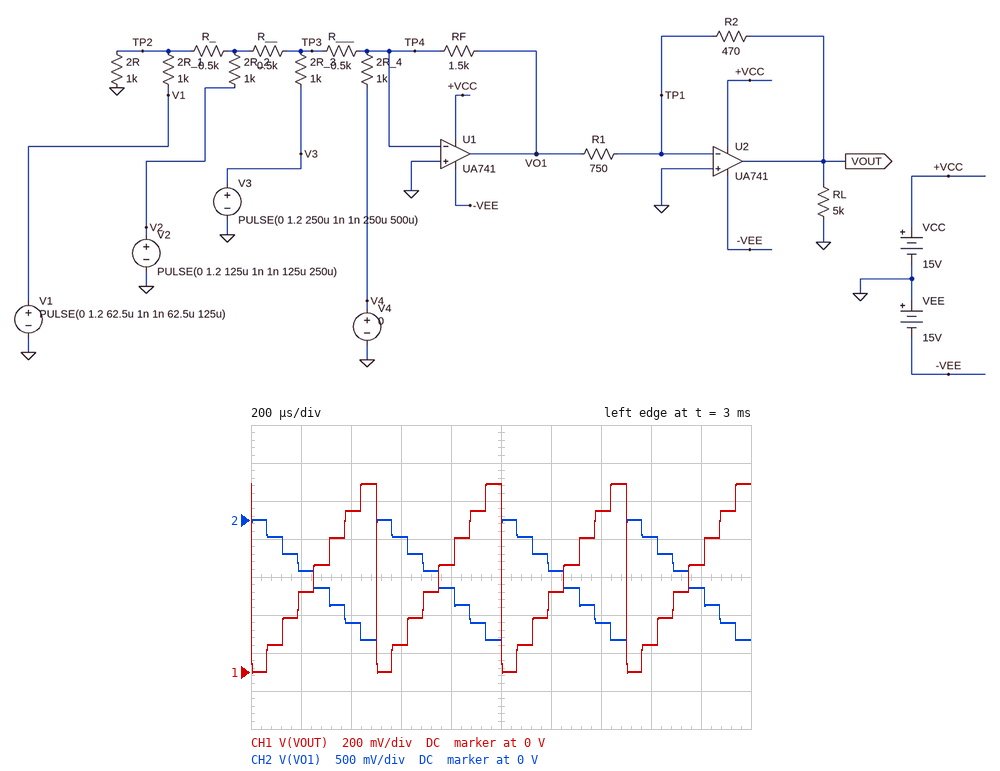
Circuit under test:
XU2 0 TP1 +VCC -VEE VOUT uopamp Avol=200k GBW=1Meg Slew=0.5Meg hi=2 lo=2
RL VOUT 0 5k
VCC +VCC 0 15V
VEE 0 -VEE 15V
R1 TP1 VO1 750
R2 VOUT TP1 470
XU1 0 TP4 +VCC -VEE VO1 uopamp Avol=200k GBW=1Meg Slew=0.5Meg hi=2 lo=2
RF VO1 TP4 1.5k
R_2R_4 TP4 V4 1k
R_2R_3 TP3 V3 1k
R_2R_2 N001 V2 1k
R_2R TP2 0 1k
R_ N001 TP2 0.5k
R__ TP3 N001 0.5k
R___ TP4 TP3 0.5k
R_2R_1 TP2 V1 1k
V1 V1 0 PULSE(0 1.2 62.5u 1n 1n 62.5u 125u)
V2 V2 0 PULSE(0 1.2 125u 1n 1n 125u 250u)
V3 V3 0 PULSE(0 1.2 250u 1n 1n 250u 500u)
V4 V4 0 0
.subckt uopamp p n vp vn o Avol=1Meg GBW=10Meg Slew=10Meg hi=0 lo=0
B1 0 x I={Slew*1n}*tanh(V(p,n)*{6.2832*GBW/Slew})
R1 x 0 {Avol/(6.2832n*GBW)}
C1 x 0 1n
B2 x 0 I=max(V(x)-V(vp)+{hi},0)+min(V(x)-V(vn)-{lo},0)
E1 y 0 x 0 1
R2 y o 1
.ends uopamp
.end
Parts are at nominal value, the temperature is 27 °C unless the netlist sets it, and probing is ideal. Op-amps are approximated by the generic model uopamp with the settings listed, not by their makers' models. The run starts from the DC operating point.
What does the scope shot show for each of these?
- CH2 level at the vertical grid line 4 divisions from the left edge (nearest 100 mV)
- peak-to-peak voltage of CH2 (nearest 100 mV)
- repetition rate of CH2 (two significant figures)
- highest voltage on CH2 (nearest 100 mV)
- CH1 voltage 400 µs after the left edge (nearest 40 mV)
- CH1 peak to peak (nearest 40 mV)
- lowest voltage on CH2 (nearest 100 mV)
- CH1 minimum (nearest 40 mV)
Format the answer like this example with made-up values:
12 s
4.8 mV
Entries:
-900 mV
1.6 V
2.0 kHz
0 V
840 mV
1.00 V
-1.6 V
0 V
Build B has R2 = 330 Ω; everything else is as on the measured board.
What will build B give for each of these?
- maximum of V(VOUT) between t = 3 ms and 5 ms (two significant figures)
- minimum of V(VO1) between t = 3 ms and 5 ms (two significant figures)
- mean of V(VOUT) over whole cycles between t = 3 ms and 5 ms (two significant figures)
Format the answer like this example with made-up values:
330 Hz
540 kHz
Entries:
690 mV
-1.6 V
350 mV
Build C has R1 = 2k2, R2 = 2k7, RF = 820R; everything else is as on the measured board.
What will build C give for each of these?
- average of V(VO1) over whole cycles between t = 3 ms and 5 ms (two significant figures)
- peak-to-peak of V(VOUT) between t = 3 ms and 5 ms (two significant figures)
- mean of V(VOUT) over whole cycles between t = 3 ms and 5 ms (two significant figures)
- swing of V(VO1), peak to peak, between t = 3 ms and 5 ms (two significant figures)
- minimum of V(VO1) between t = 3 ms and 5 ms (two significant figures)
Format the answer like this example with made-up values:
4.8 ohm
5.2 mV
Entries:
-430 mV
1.1 V
530 mV
860 mV
-860 mV
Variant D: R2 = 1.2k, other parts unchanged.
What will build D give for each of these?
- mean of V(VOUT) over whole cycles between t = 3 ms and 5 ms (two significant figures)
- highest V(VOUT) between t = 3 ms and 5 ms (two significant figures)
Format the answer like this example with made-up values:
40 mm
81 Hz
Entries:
1.3 V
2.5 V
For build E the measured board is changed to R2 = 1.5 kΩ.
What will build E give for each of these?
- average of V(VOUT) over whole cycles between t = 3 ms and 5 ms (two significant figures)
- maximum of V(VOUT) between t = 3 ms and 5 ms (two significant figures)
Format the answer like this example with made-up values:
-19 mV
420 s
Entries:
1.6 V
3.2 V
